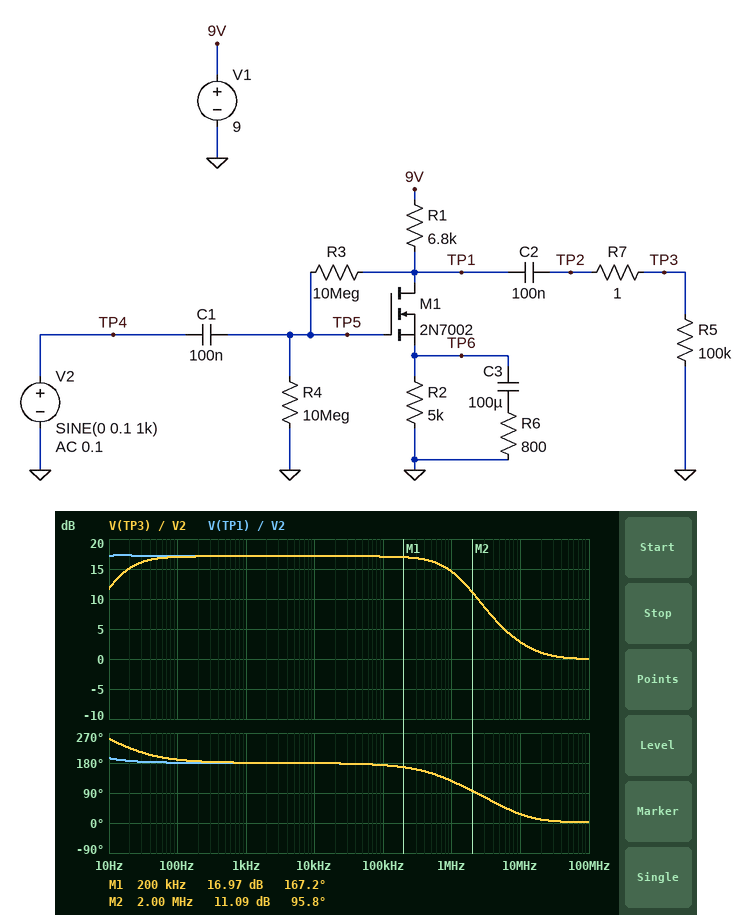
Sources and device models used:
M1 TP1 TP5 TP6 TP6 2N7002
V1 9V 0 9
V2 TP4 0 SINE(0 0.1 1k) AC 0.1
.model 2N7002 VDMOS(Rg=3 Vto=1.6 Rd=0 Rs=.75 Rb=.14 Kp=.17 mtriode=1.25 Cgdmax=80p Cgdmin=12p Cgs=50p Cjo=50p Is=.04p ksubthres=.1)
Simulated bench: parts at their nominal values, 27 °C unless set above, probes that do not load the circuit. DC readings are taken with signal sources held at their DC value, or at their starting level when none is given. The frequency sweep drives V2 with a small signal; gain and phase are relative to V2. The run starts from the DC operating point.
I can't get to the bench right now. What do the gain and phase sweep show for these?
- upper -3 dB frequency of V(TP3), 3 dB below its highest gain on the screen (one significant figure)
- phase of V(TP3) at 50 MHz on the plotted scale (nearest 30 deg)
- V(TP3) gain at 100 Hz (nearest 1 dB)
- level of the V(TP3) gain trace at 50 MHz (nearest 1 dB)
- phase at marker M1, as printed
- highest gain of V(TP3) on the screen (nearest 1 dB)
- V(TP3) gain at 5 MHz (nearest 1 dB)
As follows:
1 MHz
0 deg
17 dB
0 dB
167.2 deg
17 dB
6 dB
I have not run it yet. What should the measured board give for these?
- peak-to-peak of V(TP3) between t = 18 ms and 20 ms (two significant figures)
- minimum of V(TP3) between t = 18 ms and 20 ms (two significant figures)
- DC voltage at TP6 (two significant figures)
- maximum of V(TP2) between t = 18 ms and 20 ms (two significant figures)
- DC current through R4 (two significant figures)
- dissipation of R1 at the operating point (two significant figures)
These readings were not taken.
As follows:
1.4 V
-720 mV
1.7 V
700 mV
330 nA
820 µW
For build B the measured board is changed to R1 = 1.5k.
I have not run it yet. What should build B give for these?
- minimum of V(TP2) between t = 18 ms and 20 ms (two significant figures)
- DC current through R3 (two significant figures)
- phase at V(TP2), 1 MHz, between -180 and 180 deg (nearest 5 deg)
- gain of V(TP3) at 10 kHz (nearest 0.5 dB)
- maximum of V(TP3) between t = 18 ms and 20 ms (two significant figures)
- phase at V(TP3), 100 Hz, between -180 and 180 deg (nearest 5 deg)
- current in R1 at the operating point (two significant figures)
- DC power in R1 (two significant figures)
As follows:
-180 mV
410 nA
160 deg
5.0 dB
180 mV
-170 deg
500 µA
380 µW
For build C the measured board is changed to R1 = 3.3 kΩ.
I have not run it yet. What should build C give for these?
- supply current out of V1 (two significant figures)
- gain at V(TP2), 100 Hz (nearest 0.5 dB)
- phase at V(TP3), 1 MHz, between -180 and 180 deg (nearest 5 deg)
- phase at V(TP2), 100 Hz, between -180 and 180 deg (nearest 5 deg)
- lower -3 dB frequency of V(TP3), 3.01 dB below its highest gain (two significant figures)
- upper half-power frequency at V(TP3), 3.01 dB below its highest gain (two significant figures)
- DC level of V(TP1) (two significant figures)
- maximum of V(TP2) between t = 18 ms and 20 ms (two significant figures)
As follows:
440 µA
11.5 dB
145 deg
-170 deg
16 Hz
2.8 MHz
7.6 V
370 mV
